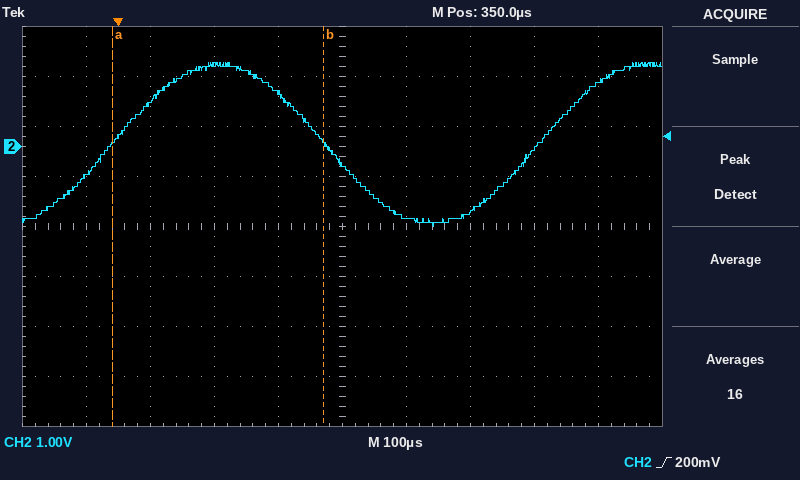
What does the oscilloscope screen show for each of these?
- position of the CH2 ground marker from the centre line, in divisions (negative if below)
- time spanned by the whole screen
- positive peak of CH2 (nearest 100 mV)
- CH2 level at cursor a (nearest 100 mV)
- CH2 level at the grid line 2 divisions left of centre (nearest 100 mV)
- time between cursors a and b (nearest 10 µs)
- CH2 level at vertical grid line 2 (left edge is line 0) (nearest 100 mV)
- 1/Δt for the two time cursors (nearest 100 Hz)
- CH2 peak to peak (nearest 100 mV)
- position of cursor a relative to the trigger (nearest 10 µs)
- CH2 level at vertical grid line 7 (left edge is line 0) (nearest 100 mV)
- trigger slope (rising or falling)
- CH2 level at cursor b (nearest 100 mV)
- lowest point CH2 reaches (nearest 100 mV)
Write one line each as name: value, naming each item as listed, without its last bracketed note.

position of the CH2 ground marker from the centre line, in divisions: +1.6 div
time spanned by the whole screen: 1 ms
positive peak of CH2: 1.7 V
CH2 level at cursor a: 100 mV
CH2 level at the grid line 2 divisions left of centre: 1.6 V
time between cursors a and b: 330 µs
CH2 level at vertical grid line 2 (left edge is line 0): 900 mV
1/Δt for the two time cursors: 3.0 kHz
CH2 peak to peak: 3.3 V
position of cursor a relative to the trigger: -10 µs
CH2 level at vertical grid line 7 (left edge is line 0): -1.3 V
trigger slope: rising
CH2 level at cursor b: 100 mV
lowest point CH2 reaches: -1.6 V
